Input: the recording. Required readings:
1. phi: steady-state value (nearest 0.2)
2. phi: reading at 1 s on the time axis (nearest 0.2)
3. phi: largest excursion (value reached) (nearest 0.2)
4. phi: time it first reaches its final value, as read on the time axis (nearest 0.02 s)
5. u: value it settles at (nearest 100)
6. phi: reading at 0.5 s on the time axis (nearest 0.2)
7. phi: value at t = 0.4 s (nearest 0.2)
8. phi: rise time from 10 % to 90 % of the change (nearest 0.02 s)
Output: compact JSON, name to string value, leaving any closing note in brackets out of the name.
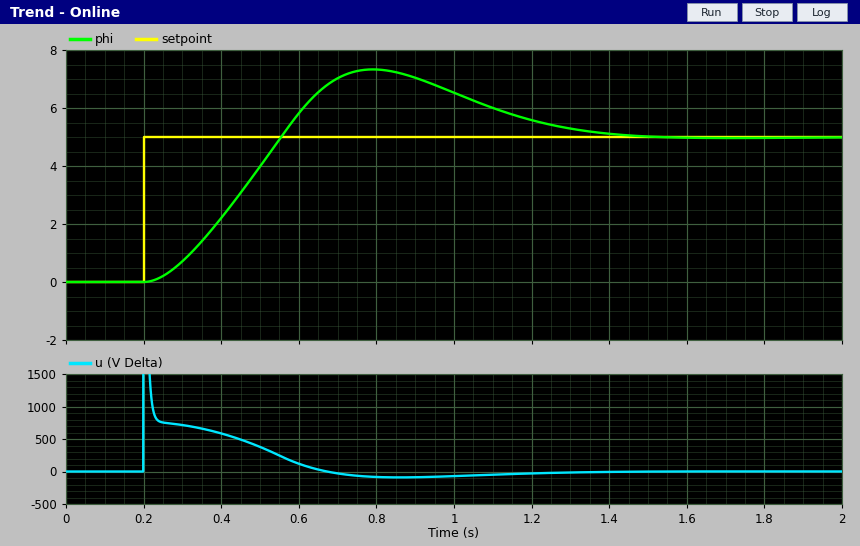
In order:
{"phi: steady-state value": "5.0", "phi: reading at 1 s on the time axis": "6.6", "phi: largest excursion (value reached)": "7.4", "phi: time it first reaches its final value, as read on the time axis": "0.56 s", "u: value it settles at": "0", "phi: reading at 0.5 s on the time axis": "4.0", "phi: value at t = 0.4 s": "2.2", "phi: rise time from 10 % to 90 % of the change": "0.24 s"}
